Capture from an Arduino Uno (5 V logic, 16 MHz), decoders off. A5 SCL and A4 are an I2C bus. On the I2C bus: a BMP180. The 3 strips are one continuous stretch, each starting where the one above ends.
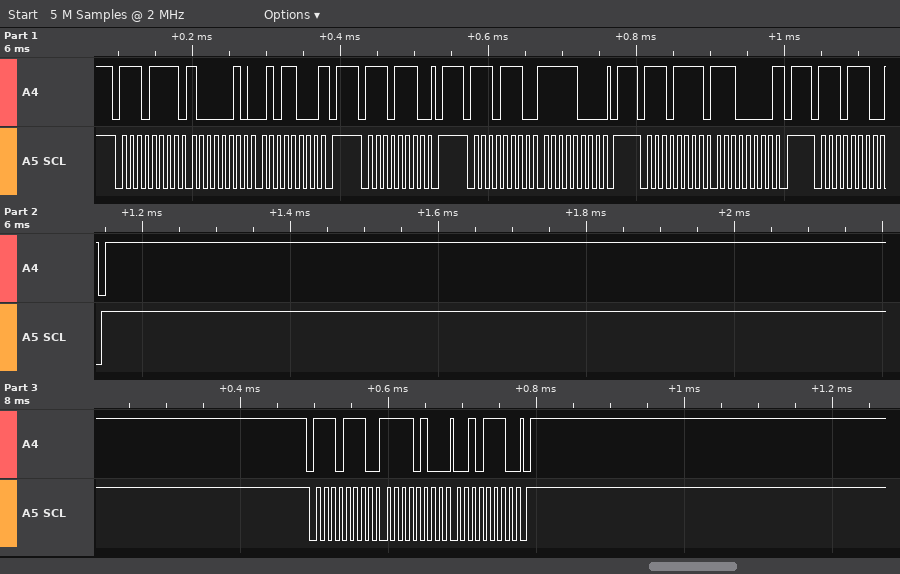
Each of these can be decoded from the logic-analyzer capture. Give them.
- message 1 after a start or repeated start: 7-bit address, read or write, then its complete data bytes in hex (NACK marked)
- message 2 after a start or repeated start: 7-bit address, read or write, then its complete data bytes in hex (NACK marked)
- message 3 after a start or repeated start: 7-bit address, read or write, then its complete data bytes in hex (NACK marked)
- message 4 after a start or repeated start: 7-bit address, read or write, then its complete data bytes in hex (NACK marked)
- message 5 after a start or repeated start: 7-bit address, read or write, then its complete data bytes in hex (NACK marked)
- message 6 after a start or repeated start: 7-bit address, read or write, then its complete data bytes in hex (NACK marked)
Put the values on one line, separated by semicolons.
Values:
0x77 read: 82 58 NACK; 0x77 write; 0x77 write: F8; 0x77 read: E0 NACK; 0x77 write; 0x77 write: F4 2E
